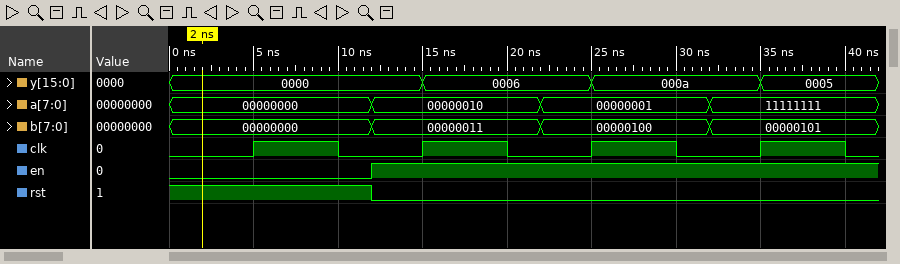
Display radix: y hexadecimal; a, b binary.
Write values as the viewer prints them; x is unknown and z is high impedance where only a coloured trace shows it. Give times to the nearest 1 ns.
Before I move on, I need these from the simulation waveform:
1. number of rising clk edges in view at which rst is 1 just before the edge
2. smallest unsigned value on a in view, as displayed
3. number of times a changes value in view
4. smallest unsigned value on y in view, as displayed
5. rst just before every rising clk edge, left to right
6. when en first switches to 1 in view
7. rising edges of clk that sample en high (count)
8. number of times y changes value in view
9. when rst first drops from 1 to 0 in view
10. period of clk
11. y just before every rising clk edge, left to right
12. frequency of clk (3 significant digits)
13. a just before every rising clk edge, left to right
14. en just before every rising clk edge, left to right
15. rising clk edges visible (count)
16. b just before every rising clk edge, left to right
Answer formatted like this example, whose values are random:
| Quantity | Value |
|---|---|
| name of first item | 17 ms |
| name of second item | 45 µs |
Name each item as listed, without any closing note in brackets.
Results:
| Quantity | Value |
|---|---|
| number of rising clk edges in view at which rst is 1 just before the edge | 1 |
| smallest unsigned value on a in view, as displayed | 00000000 |
| number of times a changes value in view | 3 |
| smallest unsigned value on y in view, as displayed | 0000 |
| rst just before every rising clk edge, left to right | 1 0 0 0 |
| when en first switches to 1 in view | 12 ns |
| rising edges of clk that sample en high | 3 |
| number of times y changes value in view | 3 |
| when rst first drops from 1 to 0 in view | 12 ns |
| period of clk | 10 ns |
| y just before every rising clk edge, left to right | 0000, 0000, 0006, 000a |
| frequency of clk | 100 MHz |
| a just before every rising clk edge, left to right | 00000000, 00000010, 00000001, 11111111 |
| en just before every rising clk edge, left to right | 0 1 1 1 |
| rising clk edges visible | 4 |
| b just before every rising clk edge, left to right | 00000000, 00000011, 00000100, 00000101 |
